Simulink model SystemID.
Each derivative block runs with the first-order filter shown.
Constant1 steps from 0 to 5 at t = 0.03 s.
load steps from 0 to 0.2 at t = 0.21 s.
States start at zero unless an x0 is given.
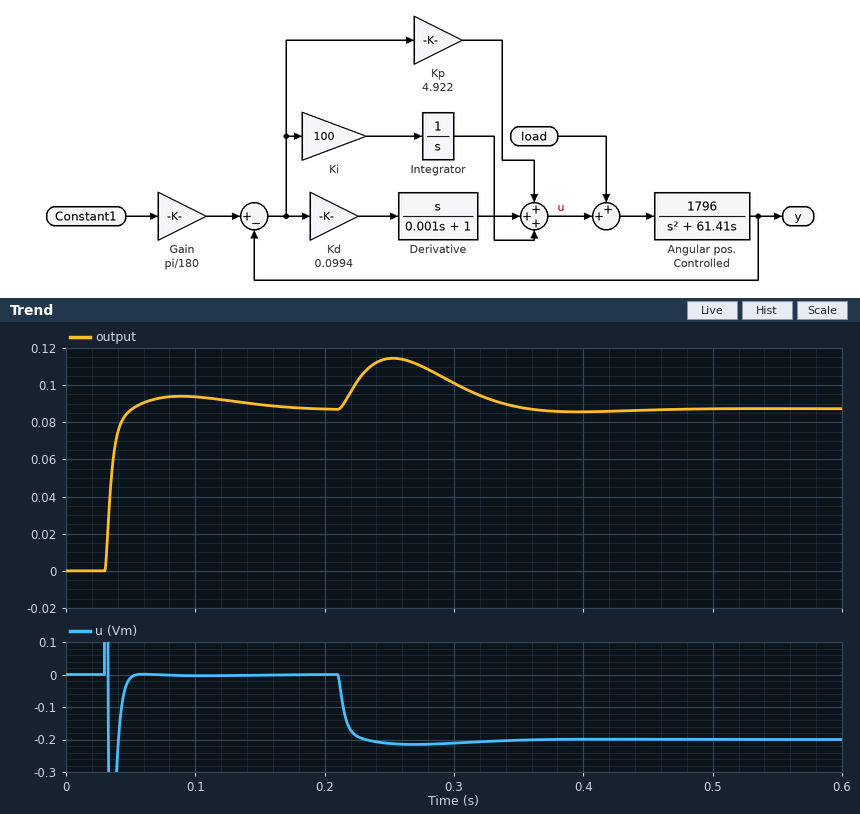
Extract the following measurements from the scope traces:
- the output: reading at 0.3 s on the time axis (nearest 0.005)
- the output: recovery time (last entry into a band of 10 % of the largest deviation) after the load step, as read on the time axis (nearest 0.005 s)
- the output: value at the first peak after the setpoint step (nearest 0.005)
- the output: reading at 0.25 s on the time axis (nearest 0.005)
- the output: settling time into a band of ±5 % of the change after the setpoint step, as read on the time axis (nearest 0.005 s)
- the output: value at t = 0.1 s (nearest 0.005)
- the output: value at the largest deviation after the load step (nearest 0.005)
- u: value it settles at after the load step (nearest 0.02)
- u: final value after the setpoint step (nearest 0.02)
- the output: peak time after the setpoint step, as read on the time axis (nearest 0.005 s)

0.100
0.340 s
0.095
0.115
0.125 s
0.095
0.115
-0.20
0.00
0.090 s
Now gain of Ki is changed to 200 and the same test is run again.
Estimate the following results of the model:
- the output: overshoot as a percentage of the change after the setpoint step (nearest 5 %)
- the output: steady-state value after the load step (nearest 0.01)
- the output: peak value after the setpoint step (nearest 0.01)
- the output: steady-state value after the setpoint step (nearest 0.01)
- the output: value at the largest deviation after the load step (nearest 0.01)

15 %
0.09
0.10
0.09
0.11
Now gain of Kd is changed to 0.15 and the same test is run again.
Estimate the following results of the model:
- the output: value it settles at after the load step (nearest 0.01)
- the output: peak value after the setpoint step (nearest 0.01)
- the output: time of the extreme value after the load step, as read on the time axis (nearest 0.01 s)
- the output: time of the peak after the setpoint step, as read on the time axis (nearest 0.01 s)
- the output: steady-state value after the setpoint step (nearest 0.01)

0.09
0.09
0.26 s
0.11 s
0.09
